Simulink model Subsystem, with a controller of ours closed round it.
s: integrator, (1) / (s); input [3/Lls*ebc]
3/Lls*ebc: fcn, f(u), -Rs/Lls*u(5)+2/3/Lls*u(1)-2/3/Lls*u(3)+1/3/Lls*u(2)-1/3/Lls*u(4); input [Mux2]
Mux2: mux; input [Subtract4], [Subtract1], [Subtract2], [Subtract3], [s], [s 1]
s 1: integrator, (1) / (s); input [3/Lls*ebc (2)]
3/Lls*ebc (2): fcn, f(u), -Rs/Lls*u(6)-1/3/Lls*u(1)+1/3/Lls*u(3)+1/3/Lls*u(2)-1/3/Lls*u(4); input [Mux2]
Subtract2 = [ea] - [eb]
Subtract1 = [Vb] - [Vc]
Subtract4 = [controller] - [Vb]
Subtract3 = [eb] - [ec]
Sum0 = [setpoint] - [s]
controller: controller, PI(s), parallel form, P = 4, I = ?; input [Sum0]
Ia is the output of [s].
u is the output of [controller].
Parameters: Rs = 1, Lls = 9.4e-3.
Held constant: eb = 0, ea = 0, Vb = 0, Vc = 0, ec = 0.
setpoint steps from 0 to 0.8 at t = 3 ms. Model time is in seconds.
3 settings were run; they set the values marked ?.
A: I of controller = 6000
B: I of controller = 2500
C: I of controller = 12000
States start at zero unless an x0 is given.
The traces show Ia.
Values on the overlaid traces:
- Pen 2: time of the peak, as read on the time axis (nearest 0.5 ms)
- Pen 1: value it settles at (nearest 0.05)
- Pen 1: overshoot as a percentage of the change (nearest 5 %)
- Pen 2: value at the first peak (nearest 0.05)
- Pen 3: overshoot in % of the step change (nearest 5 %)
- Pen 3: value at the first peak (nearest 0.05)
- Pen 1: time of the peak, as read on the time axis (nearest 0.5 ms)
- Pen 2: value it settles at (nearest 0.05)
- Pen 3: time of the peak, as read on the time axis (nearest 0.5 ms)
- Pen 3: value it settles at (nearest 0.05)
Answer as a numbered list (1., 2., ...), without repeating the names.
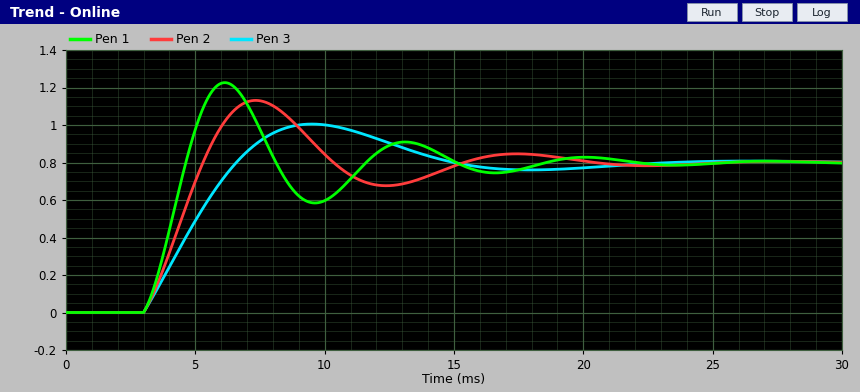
1. 7.5 ms
2. 0.80
3. 55 %
4. 1.15
5. 25 %
6. 1.00
7. 6.0 ms
8. 0.80
9. 9.5 ms
10. 0.80
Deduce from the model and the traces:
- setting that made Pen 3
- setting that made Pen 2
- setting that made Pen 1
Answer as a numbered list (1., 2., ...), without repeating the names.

1. B
2. A
3. C
